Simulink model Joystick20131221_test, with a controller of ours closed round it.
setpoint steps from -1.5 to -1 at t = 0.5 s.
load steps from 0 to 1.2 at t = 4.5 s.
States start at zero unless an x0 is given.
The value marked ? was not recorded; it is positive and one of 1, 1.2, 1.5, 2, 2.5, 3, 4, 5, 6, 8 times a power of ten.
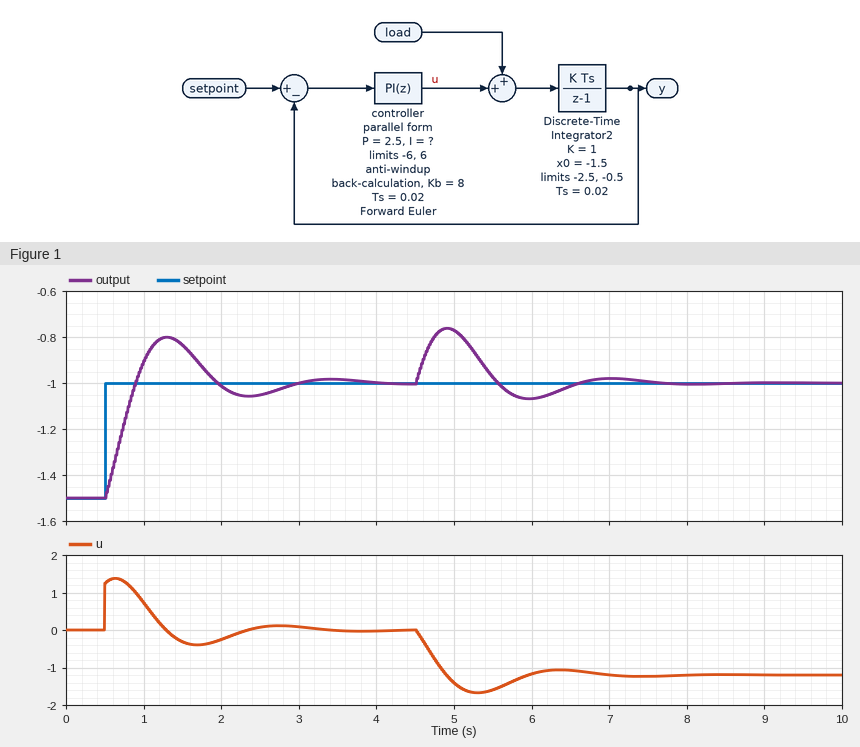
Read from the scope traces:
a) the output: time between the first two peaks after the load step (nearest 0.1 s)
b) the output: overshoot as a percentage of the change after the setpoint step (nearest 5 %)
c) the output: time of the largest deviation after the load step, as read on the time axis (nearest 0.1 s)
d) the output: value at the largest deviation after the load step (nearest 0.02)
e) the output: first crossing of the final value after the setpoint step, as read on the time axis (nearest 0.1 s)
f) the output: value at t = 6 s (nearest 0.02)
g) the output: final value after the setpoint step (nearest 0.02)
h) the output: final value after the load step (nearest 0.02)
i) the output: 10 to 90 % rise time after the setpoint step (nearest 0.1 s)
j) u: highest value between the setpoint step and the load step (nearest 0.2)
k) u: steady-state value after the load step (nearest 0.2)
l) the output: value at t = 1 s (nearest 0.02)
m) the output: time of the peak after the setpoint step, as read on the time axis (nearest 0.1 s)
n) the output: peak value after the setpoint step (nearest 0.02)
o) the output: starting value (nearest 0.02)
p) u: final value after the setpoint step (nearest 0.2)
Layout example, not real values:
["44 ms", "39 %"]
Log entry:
["2.1 s", "40 %", "4.9 s", "-0.76", "0.9 s", "-1.06", "-1.00", "-1.00", "0.3 s", "1.4", "-1.2", "-0.90", "1.3 s", "-0.80", "-1.50", "0.0"]
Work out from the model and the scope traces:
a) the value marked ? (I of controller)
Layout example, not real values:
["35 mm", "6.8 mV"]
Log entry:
["10"]
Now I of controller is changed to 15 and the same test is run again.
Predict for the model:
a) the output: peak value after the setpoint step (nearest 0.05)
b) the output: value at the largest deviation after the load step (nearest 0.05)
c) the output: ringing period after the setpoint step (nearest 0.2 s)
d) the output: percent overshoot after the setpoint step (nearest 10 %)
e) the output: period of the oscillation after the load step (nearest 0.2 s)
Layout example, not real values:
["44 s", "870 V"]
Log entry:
["-0.75", "-0.80", "1.6 s", "50 %", "1.6 s"]
